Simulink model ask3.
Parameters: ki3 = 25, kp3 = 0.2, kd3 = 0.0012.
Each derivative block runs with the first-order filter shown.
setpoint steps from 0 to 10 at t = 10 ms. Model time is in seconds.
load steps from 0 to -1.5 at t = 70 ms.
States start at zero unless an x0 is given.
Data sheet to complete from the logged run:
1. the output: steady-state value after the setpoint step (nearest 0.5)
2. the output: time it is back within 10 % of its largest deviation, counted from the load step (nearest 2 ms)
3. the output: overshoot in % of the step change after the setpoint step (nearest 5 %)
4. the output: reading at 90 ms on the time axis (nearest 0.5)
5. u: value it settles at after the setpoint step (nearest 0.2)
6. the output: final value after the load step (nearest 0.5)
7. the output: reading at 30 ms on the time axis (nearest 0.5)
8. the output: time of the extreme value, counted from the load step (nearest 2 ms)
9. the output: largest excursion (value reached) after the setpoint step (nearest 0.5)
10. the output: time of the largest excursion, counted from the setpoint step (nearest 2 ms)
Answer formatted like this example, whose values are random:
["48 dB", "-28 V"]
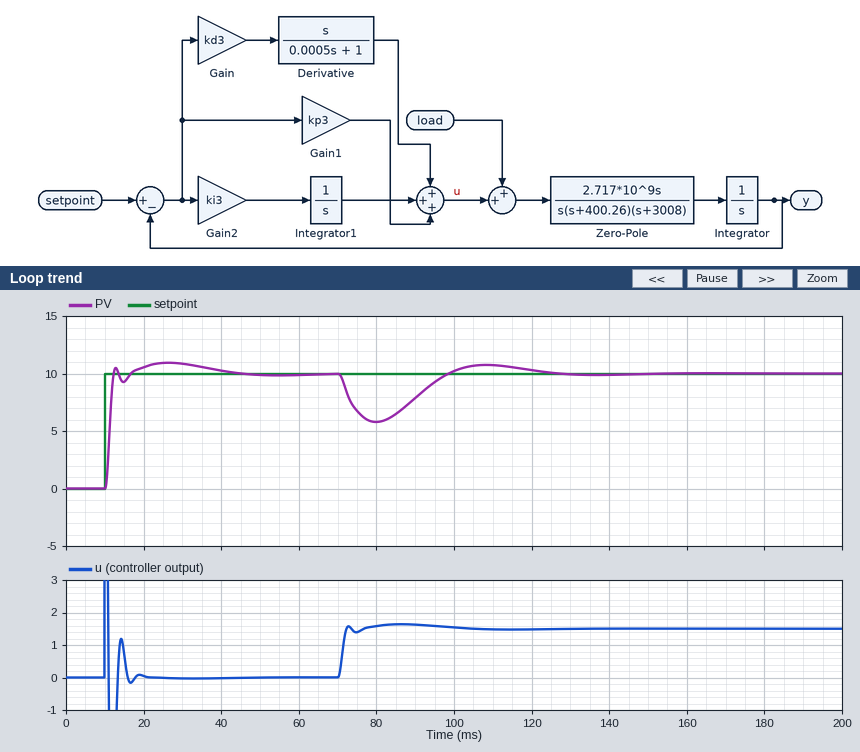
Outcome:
["10.0", "48 ms", "10 %", "8.0", "0.0", "10.0", "11.0", "10 ms", "11.0", "16 ms"]
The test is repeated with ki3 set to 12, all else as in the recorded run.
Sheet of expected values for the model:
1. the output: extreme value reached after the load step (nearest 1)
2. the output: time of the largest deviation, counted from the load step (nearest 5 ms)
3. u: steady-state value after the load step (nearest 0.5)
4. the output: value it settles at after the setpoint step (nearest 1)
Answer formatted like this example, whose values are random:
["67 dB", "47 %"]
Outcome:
["5", "15 ms", "1.5", "10"]
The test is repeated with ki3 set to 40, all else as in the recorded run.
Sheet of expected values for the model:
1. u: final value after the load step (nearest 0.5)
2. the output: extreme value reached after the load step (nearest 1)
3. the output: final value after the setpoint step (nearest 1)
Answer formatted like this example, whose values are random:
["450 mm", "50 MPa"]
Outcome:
["1.5", "6", "10"]
